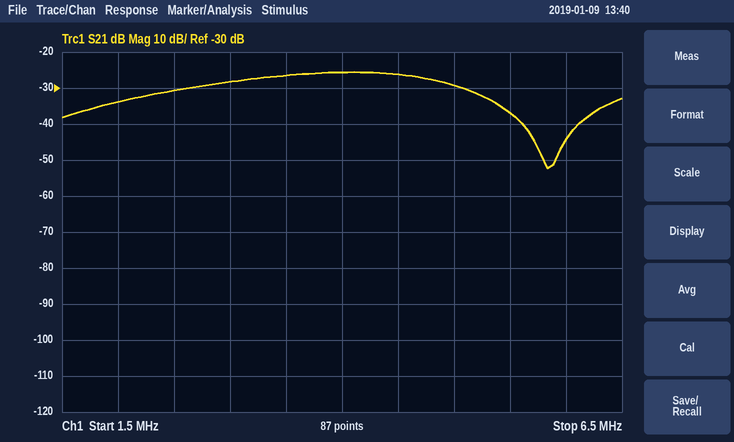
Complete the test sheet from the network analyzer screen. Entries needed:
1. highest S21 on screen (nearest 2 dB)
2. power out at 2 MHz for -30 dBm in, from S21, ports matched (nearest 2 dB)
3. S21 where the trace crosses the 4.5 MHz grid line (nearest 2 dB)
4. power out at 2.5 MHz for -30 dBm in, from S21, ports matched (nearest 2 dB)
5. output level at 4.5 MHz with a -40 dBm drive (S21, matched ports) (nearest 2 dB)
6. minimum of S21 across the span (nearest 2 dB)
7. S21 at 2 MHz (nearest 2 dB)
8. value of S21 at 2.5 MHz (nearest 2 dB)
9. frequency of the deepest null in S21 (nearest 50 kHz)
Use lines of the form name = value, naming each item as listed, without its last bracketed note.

highest S21 on screen = -26 dB
power out at 2 MHz for -30 dBm in, from S21, ports matched = -64 dBm
S21 where the trace crosses the 4.5 MHz grid line = -26 dB
power out at 2.5 MHz for -30 dBm in, from S21, ports matched = -60 dBm
output level at 4.5 MHz with a -40 dBm drive (S21, matched ports) = -66 dBm
minimum of S21 across the span = -52 dB
S21 at 2 MHz = -34 dB
value of S21 at 2.5 MHz = -30 dB
frequency of the deepest null in S21 = 5.85 MHz
